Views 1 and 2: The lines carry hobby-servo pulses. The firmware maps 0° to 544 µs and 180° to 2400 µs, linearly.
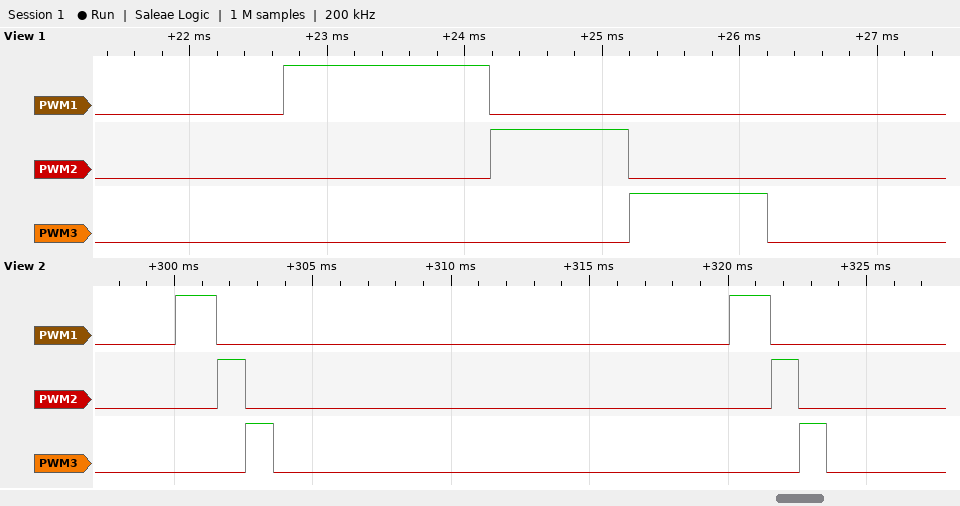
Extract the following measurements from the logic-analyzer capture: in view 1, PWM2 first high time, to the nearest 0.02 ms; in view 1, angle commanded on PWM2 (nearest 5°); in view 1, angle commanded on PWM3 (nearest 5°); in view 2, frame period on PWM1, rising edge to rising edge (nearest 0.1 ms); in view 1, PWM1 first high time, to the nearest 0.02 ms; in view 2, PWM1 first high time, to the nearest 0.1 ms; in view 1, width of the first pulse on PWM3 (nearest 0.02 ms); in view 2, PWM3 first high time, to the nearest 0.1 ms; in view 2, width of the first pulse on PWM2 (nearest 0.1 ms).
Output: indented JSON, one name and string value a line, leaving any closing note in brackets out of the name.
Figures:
{
  "in view 1, PWM2 first high time, to the nearest 0.02 ms": "1.00 ms",
  "in view 1, angle commanded on PWM2": "45°",
  "in view 1, angle commanded on PWM3": "45°",
  "in view 2, frame period on PWM1, rising edge to rising edge": "20.0 ms",
  "in view 1, PWM1 first high time, to the nearest 0.02 ms": "1.50 ms",
  "in view 2, PWM1 first high time, to the nearest 0.1 ms": "1.5 ms",
  "in view 1, width of the first pulse on PWM3": "1.00 ms",
  "in view 2, PWM3 first high time, to the nearest 0.1 ms": "1.0 ms",
  "in view 2, width of the first pulse on PWM2": "1.0 ms"
}
